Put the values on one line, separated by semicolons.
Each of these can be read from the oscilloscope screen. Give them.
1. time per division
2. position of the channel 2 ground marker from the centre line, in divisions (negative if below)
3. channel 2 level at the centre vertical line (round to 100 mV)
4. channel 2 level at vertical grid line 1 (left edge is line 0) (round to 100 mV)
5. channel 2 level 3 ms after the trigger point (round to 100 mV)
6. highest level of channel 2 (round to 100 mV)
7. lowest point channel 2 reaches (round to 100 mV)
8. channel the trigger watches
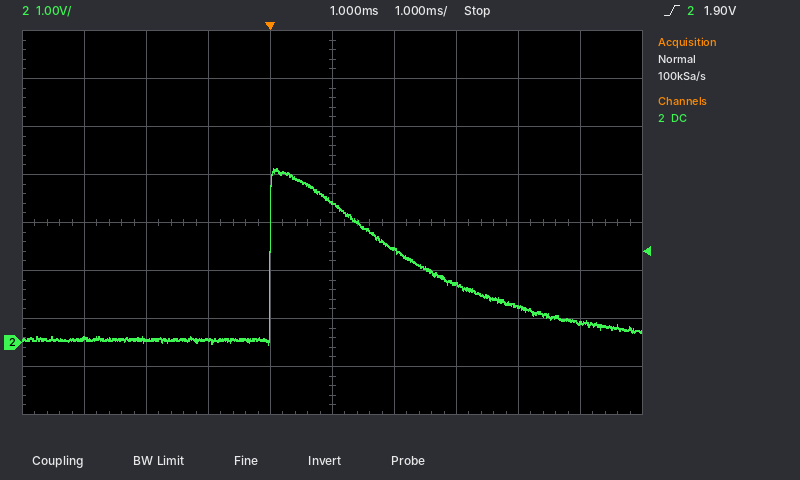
1 ms; -2.5 div; 2.9 V; 100 mV; 1.2 V; 3.6 V; 0.0 V; channel 2
